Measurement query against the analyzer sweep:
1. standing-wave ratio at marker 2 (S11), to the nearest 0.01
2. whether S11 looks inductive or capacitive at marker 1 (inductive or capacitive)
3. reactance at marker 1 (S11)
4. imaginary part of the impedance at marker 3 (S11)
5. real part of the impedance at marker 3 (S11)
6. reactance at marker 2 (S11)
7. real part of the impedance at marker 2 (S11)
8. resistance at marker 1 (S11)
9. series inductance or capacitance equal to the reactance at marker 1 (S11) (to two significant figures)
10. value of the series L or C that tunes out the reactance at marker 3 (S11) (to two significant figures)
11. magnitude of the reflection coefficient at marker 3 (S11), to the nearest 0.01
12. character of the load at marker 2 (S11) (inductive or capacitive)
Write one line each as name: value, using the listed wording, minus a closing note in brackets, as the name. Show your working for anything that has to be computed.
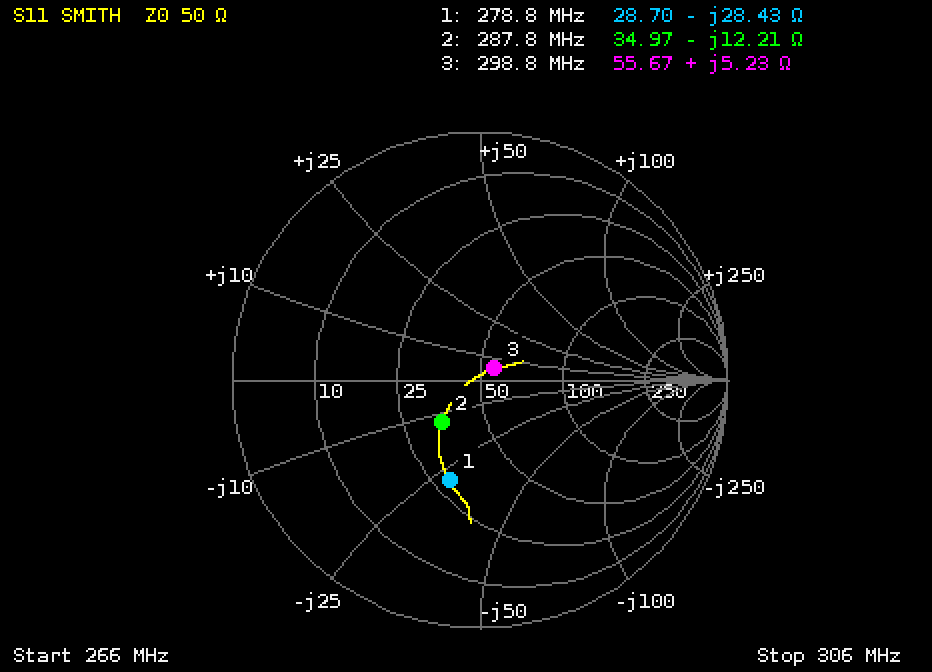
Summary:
standing-wave ratio at marker 2 (S11), to the nearest 0.01: 1.58
whether S11 looks inductive or capacitive at marker 1: capacitive
reactance at marker 1: -28.43 Ω
imaginary part of the impedance at marker 3: +5.23 Ω
real part of the impedance at marker 3: 55.67 Ω
reactance at marker 2: -12.21 Ω
real part of the impedance at marker 2: 34.97 Ω
resistance at marker 1: 28.70 Ω
series inductance or capacitance equal to the reactance at marker 1 (S11): C = 1/(2π × 278.8 MHz × 28.43 Ω) ≈ 20 pF
value of the series L or C that tunes out the reactance at marker 3 (S11): C = 1/(2π × 298.8 MHz × 5.23 Ω) ≈ 102 pF, so 100 pF to two significant figures
magnitude of the reflection coefficient at marker 3 (S11), to the nearest 0.01: 0.07
character of the load at marker 2 (S11): capacitive
